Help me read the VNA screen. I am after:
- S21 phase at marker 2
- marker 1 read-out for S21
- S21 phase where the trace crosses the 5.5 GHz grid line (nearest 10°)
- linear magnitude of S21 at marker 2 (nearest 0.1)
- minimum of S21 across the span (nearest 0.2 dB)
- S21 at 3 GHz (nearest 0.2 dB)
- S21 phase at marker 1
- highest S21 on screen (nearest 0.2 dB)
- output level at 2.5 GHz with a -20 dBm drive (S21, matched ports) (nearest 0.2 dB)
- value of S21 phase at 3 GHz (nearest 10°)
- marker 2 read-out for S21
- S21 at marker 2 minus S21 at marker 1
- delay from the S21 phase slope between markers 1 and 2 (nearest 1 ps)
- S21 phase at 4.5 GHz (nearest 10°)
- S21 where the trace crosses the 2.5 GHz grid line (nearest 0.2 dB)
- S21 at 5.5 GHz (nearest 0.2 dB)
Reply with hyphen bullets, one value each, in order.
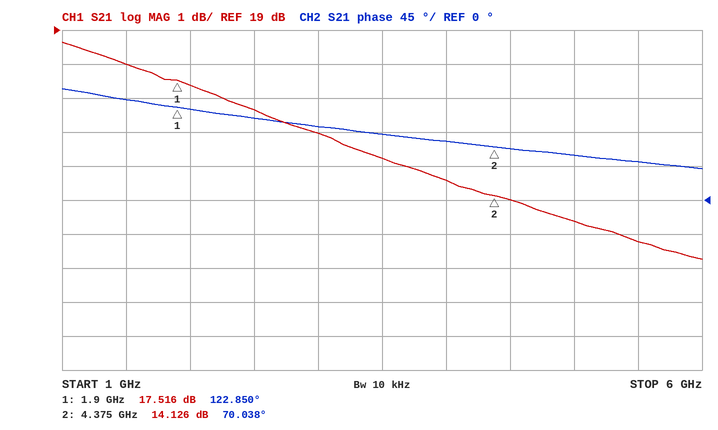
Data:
- 70.038°
- 17.516 dB
- 50°
- 5.1
- 12.2 dB
- 16.0 dB
- 122.850°
- 18.6 dB
- -3.4 dBm
- 100°
- 14.126 dB
- -3.390 dB
- 59 ps
- 70°
- 16.6 dB
- 12.8 dB
